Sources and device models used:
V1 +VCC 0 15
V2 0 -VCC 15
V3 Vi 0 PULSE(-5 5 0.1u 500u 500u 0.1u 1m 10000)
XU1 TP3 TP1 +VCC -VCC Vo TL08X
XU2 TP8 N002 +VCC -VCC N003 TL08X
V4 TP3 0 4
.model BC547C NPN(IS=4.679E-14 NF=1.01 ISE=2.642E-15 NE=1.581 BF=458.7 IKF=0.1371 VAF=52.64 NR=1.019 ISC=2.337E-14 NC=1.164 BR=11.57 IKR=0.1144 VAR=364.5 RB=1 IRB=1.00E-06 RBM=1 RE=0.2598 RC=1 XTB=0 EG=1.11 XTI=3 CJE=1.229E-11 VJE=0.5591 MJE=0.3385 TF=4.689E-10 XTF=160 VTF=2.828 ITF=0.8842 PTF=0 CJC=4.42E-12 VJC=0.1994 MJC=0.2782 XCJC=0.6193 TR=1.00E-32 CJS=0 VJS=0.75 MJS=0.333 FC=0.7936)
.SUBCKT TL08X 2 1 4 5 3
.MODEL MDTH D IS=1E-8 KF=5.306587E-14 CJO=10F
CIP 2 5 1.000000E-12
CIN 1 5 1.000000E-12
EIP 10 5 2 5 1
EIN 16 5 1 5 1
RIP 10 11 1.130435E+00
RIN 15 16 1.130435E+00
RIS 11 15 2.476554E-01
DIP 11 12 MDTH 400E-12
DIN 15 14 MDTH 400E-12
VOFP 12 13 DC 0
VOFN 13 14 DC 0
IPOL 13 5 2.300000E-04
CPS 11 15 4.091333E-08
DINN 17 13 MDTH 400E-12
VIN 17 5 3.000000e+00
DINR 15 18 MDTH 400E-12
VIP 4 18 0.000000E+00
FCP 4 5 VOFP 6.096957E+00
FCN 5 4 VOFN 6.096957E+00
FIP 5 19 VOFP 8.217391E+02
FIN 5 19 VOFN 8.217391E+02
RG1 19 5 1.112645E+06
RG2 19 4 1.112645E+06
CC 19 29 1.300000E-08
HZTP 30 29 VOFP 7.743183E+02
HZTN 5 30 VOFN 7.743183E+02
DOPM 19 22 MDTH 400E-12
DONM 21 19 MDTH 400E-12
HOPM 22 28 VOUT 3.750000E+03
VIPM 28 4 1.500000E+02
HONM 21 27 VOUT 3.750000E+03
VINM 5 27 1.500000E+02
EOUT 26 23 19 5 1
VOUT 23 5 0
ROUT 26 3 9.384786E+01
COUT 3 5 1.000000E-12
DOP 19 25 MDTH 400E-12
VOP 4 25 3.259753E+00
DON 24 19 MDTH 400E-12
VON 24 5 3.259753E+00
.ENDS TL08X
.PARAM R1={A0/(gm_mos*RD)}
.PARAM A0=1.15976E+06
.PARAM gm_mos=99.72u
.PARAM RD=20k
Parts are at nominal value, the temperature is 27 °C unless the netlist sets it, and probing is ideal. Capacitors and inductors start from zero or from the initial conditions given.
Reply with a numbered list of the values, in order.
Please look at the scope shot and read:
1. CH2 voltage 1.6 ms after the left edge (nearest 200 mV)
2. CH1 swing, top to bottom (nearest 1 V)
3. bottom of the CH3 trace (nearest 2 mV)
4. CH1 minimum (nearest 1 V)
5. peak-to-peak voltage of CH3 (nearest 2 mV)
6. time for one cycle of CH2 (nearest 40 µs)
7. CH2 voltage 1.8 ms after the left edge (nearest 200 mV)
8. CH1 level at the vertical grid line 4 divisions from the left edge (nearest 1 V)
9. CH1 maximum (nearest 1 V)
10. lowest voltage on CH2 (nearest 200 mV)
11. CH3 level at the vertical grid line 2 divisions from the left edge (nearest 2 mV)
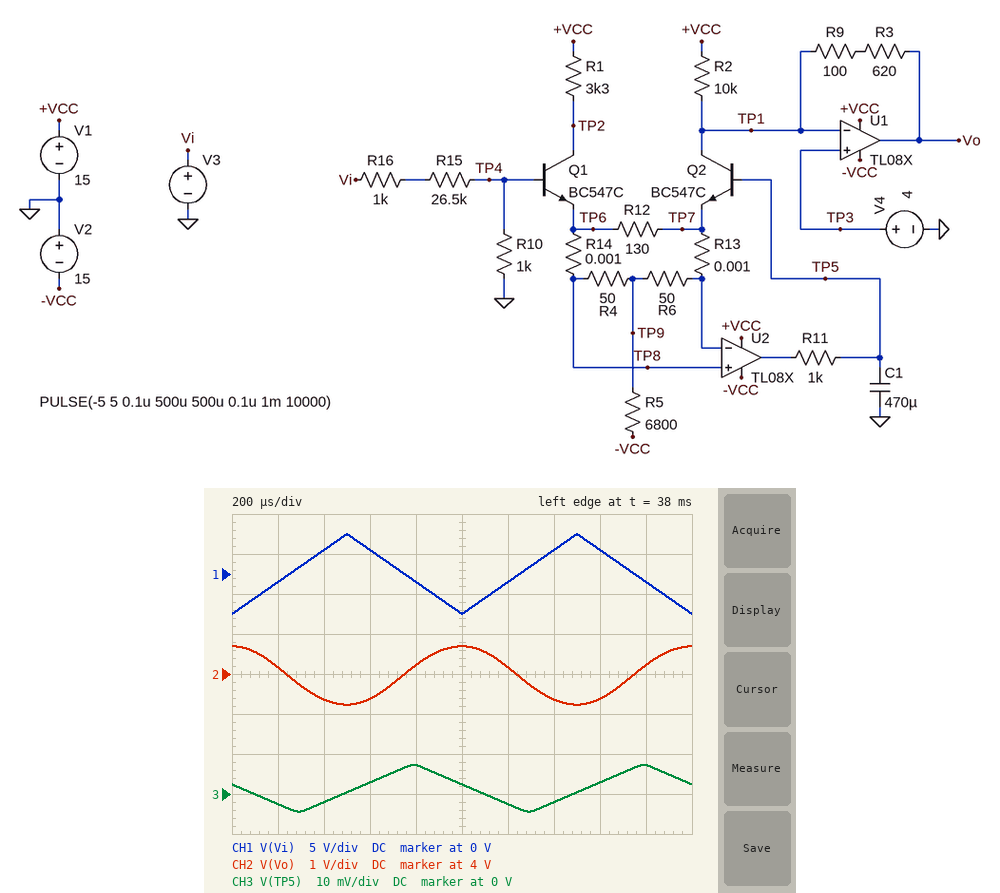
1. 3.4 V
2. 10 V
3. -4 mV
4. -5 V
5. 12 mV
6. 1.00 ms
7. 4.2 V
8. -1 V
9. 5 V
10. 3.2 V
11. -2 mV
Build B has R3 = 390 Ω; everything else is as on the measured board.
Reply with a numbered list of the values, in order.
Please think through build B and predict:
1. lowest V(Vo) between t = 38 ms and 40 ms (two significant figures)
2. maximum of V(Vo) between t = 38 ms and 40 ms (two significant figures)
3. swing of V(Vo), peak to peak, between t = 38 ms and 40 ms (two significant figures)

1. 3.5 V
2. 4.5 V
3. 1.0 V
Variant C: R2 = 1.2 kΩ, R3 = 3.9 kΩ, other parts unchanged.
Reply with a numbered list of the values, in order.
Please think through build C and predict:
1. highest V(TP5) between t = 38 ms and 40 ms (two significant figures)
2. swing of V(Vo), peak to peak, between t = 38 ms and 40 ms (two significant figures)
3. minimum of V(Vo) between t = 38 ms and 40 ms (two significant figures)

1. 5.6 mV
2. 43 mV
3. -12 V
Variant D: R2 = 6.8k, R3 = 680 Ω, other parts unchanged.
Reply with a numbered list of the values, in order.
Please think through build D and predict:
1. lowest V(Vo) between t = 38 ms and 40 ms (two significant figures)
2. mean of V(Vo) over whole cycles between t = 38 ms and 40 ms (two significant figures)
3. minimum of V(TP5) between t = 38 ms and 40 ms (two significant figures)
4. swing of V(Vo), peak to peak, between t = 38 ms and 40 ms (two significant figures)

1. 2.8 V
2. 3.6 V
3. -4.4 mV
4. 1.6 V
